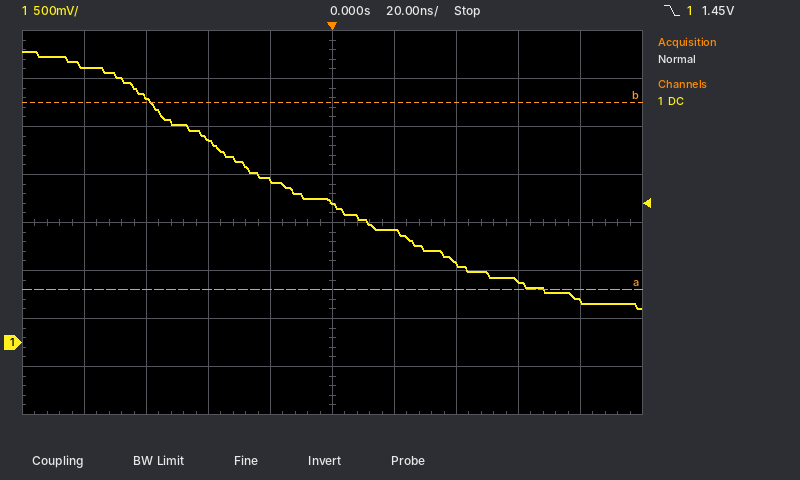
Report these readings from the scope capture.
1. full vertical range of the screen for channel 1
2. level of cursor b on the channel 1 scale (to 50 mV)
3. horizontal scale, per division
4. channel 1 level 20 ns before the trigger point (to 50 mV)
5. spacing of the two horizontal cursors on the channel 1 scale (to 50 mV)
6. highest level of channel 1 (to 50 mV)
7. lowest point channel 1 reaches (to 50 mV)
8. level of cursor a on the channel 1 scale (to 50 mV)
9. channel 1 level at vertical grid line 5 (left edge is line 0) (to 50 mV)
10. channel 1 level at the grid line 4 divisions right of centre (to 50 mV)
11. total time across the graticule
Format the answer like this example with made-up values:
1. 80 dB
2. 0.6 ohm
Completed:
1. 4 V
2. 2.50 V
3. 20 ns
4. 1.70 V
5. 1.95 V
6. 3.05 V
7. 350 mV
8. 550 mV
9. 1.45 V
10. 450 mV
11. 200 ns
